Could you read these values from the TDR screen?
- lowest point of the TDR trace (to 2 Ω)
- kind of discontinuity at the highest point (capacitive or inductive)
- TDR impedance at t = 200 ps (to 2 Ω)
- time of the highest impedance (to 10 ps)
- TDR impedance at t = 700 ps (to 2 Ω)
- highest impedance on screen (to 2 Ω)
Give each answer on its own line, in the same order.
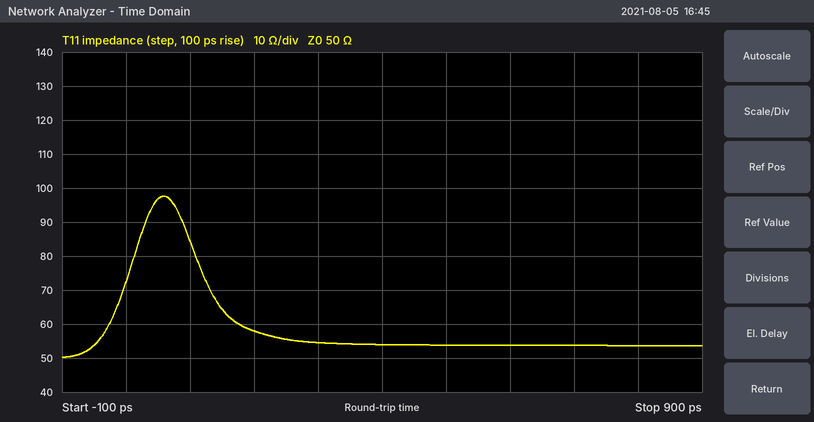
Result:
50 Ω
inductive
58 Ω
60 ps
54 Ω
98 Ω
